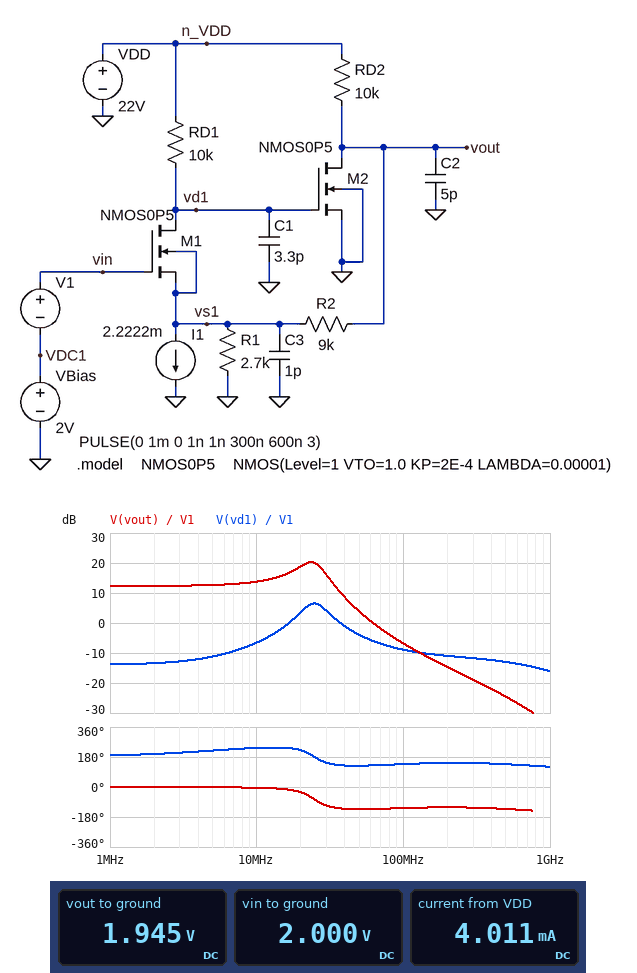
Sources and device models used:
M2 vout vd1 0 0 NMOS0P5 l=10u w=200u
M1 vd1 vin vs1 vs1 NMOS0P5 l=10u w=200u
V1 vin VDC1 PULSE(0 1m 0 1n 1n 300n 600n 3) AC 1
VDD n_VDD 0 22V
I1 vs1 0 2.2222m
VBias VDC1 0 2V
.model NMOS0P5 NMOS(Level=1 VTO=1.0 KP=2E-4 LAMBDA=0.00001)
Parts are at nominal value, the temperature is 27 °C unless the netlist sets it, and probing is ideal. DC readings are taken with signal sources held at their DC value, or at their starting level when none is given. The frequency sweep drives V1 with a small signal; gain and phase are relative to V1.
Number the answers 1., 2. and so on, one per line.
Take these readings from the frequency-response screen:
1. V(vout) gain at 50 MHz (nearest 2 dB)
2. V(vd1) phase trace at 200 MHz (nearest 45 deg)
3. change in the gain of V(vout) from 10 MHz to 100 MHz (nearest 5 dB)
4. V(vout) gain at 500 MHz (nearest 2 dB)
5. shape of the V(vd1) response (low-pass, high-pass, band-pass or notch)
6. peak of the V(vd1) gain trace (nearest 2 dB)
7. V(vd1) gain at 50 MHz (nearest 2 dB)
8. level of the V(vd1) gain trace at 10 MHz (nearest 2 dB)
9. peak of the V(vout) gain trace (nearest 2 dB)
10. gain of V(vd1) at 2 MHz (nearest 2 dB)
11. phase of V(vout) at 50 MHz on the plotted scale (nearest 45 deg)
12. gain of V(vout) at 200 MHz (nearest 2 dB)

1. 4 dB
2. 135 deg
3. -20 dB
4. -24 dB
5. band-pass
6. 6 dB
7. -4 dB
8. -6 dB
9. 20 dB
10. -14 dB
11. -135 deg
12. -14 dB
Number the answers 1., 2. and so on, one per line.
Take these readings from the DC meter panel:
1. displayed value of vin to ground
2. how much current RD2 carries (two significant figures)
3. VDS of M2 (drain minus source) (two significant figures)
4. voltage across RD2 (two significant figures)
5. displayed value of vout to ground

1. 2.000 V
2. 2.0 mA
3. 1.9 V
4. 20 V
5. 1.945 V
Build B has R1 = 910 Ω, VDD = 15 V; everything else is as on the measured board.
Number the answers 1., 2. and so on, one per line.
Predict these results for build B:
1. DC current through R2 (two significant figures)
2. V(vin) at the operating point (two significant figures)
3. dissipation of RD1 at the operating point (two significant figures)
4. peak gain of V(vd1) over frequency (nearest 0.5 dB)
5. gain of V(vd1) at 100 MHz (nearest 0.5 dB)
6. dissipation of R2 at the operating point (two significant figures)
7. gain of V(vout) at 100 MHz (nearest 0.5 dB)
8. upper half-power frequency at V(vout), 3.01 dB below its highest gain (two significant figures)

1. 790 µA
2. 2.0 V
3. 21 mW
4. -2.0 dB
5. -13.0 dB
6. 5.6 mW
7. -38.5 dB
8. 32 MHz
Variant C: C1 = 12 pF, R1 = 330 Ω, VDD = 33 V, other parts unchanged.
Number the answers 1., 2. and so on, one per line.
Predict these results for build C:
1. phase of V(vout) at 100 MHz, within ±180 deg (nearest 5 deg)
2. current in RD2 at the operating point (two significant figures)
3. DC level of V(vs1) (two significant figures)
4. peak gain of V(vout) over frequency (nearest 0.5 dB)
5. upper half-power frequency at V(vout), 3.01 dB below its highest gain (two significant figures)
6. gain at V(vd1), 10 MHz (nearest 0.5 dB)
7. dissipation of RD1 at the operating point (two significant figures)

1. -50 deg
2. 3.3 mA
3. -30 mV
4. -18.0 dB
5. 1.3 MHz
6. 7.5 dB
7. 45 mW
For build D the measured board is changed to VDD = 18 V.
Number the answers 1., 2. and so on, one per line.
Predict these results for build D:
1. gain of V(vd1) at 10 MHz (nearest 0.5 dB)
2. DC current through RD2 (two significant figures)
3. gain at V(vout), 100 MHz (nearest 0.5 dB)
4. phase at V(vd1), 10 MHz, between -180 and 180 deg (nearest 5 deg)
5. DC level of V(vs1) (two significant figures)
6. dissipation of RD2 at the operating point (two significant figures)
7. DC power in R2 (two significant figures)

1. -1.5 dB
2. 1.2 mA
3. -11.5 dB
4. -135 deg
5. 93 mV
6. 15 mW
7. 3.4 mW
